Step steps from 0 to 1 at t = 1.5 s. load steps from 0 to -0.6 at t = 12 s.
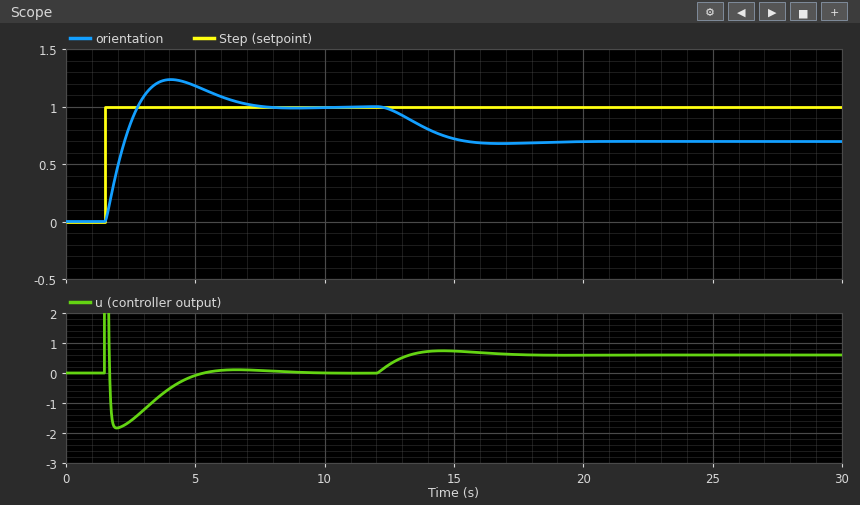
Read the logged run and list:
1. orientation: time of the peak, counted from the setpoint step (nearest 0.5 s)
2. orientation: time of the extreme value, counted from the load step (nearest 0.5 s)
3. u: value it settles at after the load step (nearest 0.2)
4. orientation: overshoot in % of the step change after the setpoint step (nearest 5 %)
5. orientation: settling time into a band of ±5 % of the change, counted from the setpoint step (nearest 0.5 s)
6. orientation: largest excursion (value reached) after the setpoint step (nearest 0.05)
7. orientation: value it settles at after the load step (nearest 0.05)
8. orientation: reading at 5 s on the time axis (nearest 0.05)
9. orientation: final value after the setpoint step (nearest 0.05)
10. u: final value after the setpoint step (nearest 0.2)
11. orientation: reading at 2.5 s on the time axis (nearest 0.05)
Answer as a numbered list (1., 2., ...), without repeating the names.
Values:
1. 2.5 s
2. 5.0 s
3. 0.6
4. 25 %
5. 5.0 s
6. 1.25
7. 0.70
8. 1.20
9. 1.00
10. 0.0
11. 0.85
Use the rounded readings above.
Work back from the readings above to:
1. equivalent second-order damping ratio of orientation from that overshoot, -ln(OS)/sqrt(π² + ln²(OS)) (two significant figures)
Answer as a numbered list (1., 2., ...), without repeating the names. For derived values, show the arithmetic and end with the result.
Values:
1. ln(0.25) = -1.386; 1.386 / sqrt(9.870 + 1.922) = 0.40
